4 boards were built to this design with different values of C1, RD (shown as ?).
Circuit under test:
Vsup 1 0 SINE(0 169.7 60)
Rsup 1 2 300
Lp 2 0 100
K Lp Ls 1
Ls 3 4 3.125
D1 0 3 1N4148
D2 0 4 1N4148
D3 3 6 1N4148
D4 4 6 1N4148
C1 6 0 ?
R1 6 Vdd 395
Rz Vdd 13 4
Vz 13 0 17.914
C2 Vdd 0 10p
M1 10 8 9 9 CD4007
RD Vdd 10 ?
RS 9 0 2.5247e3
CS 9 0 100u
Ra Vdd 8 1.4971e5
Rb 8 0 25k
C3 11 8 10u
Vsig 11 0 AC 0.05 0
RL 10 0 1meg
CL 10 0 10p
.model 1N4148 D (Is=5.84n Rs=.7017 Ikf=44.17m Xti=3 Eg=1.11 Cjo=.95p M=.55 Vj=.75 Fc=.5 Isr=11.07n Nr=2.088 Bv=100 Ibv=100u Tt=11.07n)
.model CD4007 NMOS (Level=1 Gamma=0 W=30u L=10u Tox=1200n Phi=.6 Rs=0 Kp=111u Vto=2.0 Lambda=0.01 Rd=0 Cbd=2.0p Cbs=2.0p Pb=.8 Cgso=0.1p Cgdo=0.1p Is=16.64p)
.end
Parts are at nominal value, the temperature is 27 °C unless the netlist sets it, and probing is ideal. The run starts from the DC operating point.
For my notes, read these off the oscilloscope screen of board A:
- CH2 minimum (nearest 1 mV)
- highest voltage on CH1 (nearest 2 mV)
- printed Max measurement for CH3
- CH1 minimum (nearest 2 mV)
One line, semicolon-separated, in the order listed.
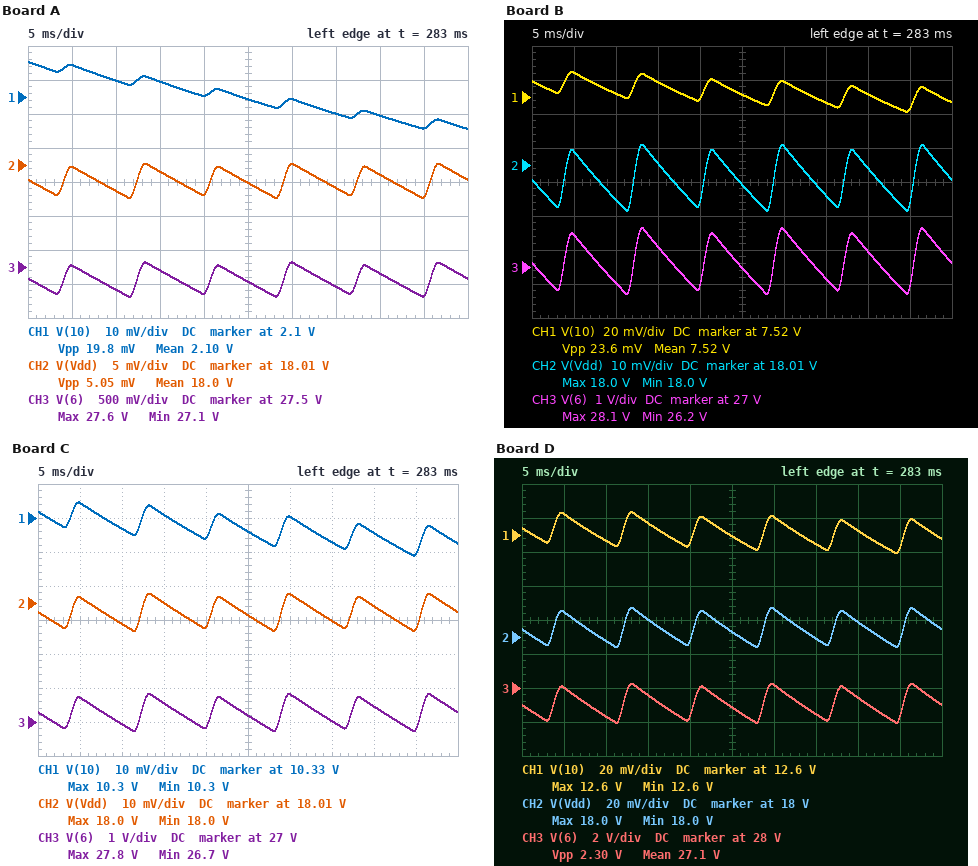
18.005 V; 2.110 V; 27.6 V; 2.090 V
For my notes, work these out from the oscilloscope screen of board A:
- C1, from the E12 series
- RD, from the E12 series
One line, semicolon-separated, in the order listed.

330 µF; 390 kΩ
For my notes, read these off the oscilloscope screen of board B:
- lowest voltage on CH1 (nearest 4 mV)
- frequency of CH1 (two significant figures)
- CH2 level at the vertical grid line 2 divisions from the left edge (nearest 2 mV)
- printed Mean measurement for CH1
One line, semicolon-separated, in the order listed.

7.512 V; 120 Hz; 18.000 V; 7.52 V
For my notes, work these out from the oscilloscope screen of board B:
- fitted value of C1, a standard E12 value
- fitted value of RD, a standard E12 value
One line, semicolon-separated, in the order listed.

82 µF; 220 kΩ
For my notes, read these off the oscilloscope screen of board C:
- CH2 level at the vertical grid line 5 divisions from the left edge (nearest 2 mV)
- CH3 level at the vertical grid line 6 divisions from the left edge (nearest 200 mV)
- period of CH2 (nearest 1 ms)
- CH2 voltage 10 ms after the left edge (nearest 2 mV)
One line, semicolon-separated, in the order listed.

18.006 V; 27.8 V; 8 ms; 18.004 V
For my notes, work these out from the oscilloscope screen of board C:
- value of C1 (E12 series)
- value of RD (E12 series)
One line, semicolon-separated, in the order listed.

150 µF; 150 kΩ
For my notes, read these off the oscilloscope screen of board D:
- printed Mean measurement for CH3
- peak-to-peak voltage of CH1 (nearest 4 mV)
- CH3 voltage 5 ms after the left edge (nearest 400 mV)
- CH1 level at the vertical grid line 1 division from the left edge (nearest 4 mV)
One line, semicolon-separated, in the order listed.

27.1 V; 24 mV; 28.0 V; 12.612 V
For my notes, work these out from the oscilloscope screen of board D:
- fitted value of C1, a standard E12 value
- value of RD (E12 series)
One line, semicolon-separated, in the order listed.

68 µF; 100 kΩ
